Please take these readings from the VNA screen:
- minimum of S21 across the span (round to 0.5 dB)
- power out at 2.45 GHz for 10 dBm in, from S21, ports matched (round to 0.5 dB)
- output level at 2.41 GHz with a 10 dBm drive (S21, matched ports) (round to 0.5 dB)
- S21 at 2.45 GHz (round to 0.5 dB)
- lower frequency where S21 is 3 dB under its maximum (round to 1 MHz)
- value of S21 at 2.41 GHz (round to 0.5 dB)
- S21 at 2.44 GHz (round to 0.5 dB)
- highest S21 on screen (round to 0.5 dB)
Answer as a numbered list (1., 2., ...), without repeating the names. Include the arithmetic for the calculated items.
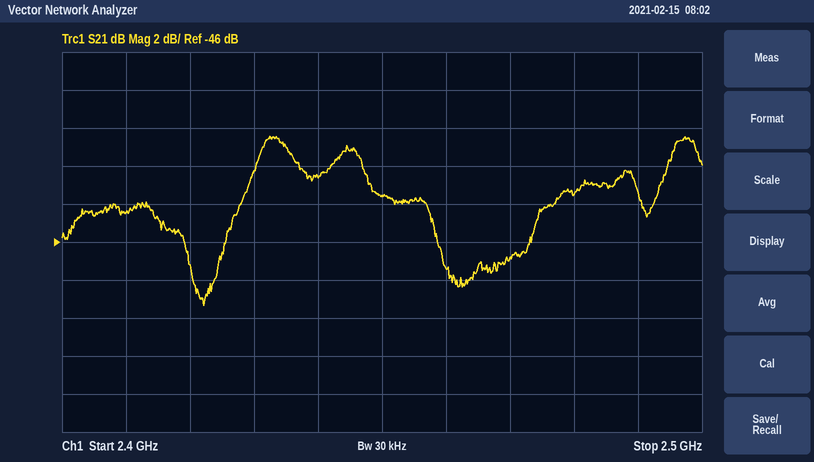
1. -49.5 dB
2. 10 dBm + (-43.5 dB) = -33.5 dBm
3. 10 dBm + (-44.5 dB) = -34.5 dBm
4. -43.5 dB
5. 2.429 GHz
6. -44.5 dB
7. -42.5 dB
8. -40.5 dB
